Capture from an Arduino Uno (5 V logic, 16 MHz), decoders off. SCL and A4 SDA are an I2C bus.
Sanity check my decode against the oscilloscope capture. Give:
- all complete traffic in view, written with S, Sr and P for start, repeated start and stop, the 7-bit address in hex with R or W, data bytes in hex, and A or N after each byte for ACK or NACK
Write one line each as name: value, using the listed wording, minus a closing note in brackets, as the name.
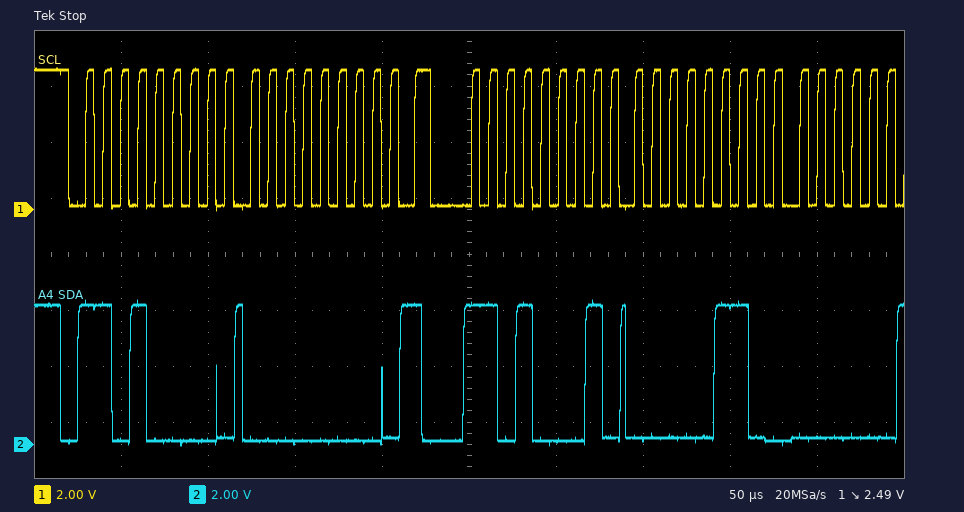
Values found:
all complete traffic in view, written with S, Sr and P for start, repeated start and stop, the 7-bit address in hex with R or W, data bytes in hex, and A or N after each byte for ACK or NACK: S 68W A 00 A Sr 68R A 06 A
